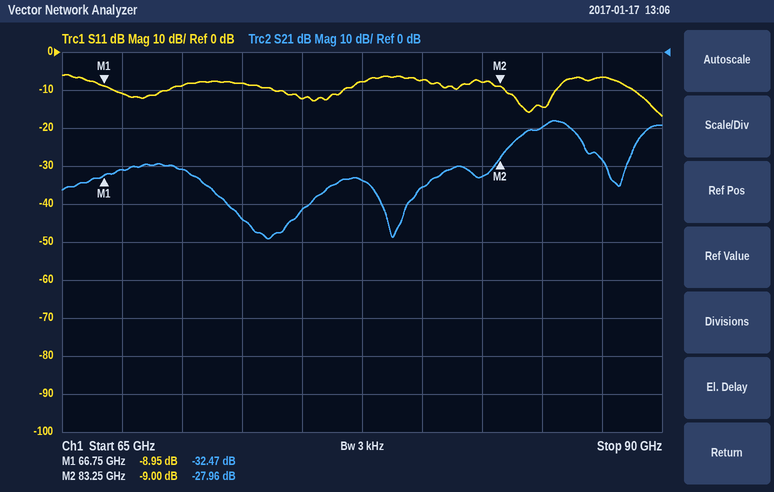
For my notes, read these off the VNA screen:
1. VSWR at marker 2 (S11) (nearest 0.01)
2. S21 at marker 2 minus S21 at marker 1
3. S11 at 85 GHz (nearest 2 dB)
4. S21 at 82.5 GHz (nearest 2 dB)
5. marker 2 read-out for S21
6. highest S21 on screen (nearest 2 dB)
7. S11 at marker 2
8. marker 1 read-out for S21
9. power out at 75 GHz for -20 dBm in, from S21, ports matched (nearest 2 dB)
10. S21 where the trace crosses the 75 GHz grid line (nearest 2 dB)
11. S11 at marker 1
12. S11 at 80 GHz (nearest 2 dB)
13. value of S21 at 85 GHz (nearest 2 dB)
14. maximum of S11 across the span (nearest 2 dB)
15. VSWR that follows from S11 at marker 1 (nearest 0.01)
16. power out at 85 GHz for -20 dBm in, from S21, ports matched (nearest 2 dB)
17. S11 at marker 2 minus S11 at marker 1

2.10
4.51 dB
-14 dB
-32 dB
-27.96 dB
-18 dB
-9.00 dB
-32.47 dB
-62 dBm
-42 dB
-8.95 dB
-8 dB
-20 dB
-6 dB
2.11
-40 dBm
-0.05 dB
